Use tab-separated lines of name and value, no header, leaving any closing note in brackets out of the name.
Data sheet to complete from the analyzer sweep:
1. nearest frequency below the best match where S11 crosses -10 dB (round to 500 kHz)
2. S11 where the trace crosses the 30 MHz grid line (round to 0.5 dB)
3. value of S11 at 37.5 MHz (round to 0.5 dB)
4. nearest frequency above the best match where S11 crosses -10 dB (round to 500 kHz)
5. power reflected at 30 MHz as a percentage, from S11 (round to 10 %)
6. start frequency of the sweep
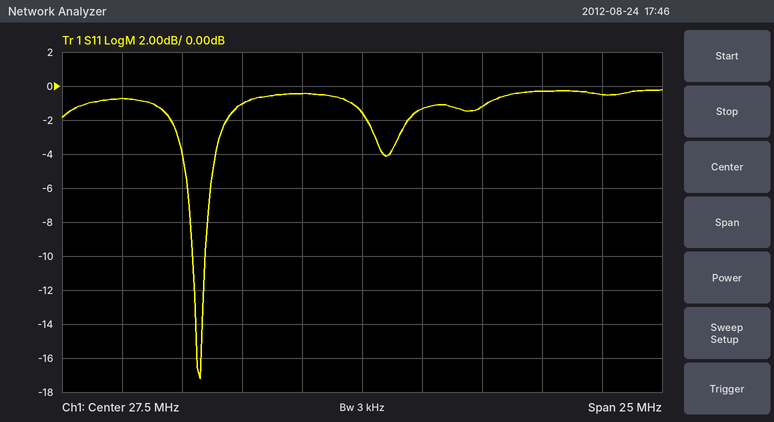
nearest frequency below the best match where S11 crosses -10 dB	20.5 MHz
S11 where the trace crosses the 30 MHz grid line	-1.5 dB
value of S11 at 37.5 MHz	-0.5 dB
nearest frequency above the best match where S11 crosses -10 dB	21.0 MHz
power reflected at 30 MHz as a percentage, from S11	70 %
start frequency of the sweep	15 MHz
